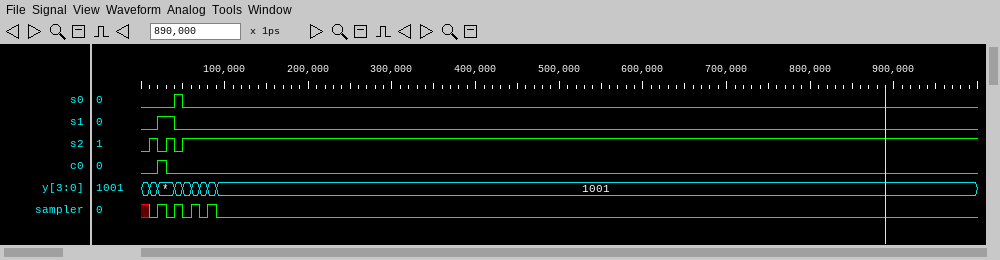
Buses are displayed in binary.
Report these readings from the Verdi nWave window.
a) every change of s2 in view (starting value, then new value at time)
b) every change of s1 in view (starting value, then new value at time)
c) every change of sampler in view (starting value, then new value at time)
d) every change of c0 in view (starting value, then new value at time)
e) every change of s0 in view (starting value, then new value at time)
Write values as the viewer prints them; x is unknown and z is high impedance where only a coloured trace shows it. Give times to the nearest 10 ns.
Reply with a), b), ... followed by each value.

a) 0, 1 at 10 ns, 0 at 20 ns, 1 at 30 ns, 0 at 40 ns, 1 at 50 ns
b) 0, 1 at 20 ns, 0 at 40 ns
c) x, 0 at 10 ns, 1 at 20 ns, 0 at 30 ns, 1 at 40 ns, 0 at 50 ns, 1 at 60 ns, 0 at 70 ns, 1 at 80 ns, 0 at 90 ns
d) 0, 1 at 20 ns, 0 at 30 ns
e) 0, 1 at 40 ns, 0 at 50 ns
